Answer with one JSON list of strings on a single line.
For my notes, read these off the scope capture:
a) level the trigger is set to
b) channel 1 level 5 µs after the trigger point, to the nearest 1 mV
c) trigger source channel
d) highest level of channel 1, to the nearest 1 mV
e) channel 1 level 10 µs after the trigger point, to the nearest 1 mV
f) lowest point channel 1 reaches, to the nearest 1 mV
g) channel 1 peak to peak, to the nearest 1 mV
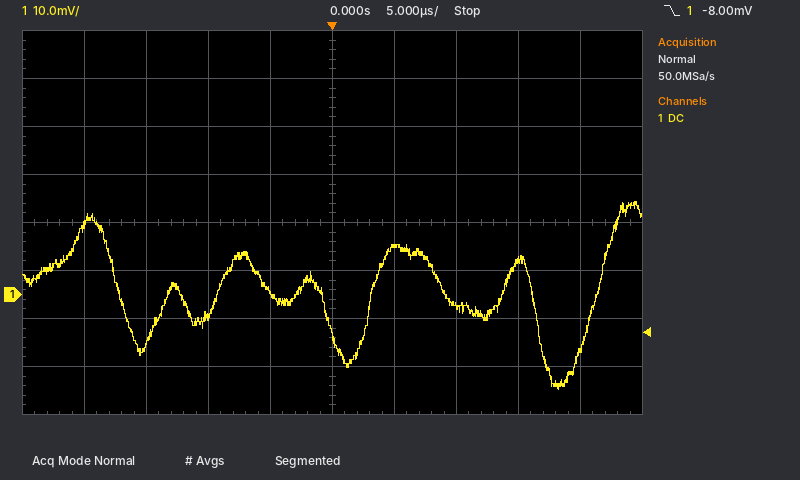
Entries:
["-8.00 mV", "10 mV", "channel 1", "19 mV", "-2 mV", "-20 mV", "39 mV"]
